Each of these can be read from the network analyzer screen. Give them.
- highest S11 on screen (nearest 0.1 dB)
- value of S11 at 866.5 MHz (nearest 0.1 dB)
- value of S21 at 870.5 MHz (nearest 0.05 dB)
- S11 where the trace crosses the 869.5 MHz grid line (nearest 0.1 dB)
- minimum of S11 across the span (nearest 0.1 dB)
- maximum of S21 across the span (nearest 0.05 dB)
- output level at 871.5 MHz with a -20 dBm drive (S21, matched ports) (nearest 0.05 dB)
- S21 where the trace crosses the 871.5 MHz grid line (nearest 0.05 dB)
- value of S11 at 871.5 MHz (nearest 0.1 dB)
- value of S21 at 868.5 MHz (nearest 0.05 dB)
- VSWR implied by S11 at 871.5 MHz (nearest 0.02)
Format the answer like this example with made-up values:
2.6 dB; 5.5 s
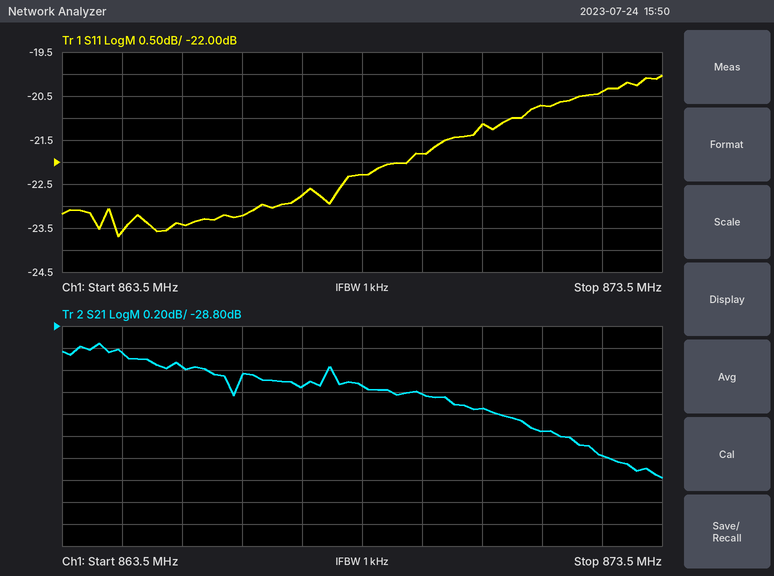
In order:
-20.0 dB; -23.2 dB; -29.55 dB; -21.8 dB; -23.7 dB; -28.95 dB; -49.75 dBm; -29.75 dB; -20.7 dB; -29.35 dB; 1.20
